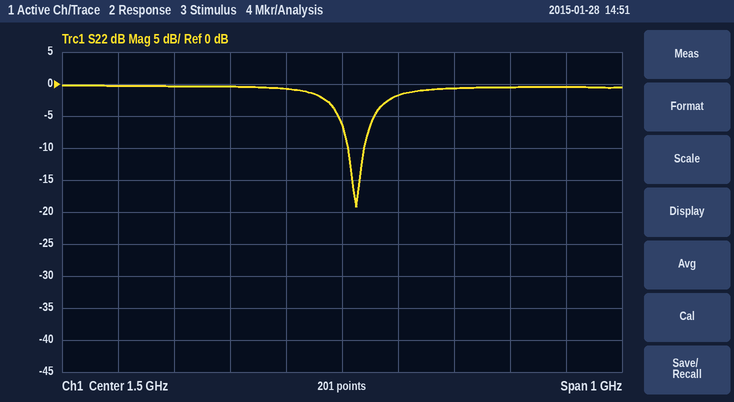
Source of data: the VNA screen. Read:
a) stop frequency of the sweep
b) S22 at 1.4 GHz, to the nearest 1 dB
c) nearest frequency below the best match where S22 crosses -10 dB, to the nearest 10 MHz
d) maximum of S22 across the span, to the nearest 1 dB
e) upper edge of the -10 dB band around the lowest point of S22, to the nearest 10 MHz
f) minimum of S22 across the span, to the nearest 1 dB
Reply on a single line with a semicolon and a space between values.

2 GHz; -1 dB; 1.51 GHz; 0 dB; 1.54 GHz; -19 dB
